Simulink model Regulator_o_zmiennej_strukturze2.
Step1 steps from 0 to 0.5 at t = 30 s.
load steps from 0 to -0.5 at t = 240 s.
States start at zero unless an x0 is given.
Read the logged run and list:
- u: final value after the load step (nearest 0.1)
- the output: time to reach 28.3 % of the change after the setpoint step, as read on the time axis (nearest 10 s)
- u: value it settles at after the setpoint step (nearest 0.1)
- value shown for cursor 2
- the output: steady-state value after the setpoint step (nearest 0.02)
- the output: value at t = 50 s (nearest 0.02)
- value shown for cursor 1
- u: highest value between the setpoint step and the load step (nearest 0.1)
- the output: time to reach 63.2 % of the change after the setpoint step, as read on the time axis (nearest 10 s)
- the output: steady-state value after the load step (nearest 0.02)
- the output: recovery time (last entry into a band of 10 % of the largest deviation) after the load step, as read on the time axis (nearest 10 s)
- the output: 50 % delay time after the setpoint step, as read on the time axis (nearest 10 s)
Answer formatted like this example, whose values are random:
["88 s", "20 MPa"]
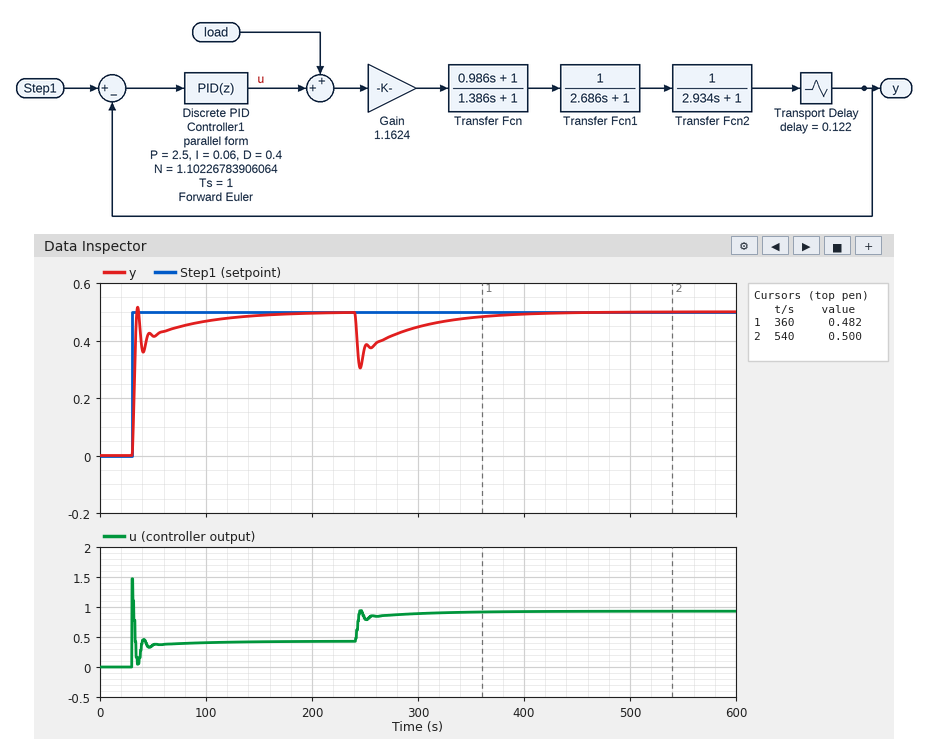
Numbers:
["0.9", "30 s", "0.4", "0.500", "0.50", "0.42", "0.482", "1.5", "30 s", "0.50", "350 s", "30 s"]
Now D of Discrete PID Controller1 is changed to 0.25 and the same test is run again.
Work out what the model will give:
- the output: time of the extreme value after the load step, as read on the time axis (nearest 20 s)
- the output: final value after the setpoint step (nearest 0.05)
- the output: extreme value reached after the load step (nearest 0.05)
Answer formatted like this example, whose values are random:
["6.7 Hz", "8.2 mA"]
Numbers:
["240 s", "0.50", "0.30"]
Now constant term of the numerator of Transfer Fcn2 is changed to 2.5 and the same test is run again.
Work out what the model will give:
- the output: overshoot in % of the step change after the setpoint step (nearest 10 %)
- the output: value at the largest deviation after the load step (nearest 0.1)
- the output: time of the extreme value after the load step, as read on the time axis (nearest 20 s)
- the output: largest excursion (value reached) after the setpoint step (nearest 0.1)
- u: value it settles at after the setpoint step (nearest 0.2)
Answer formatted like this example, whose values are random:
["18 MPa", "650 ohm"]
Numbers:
["60 %", "0.2", "240 s", "0.8", "0.2"]
